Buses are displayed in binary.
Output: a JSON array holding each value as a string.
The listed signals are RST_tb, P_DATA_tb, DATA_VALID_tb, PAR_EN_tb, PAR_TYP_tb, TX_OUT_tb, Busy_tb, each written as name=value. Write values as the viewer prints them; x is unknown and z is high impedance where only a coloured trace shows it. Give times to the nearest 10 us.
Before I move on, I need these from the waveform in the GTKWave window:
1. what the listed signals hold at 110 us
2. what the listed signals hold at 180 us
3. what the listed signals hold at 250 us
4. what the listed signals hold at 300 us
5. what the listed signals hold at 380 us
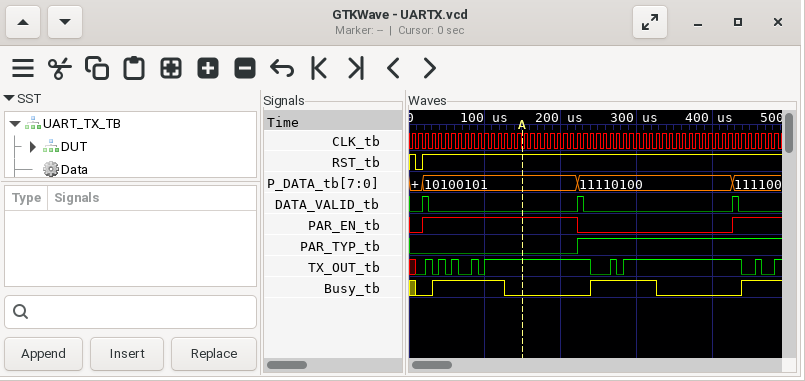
["RST_tb=1, P_DATA_tb=10100101, DATA_VALID_tb=0, PAR_EN_tb=1, PAR_TYP_tb=0, TX_OUT_tb=1, Busy_tb=1", "RST_tb=1, P_DATA_tb=10100101, DATA_VALID_tb=0, PAR_EN_tb=1, PAR_TYP_tb=0, TX_OUT_tb=1, Busy_tb=0", "RST_tb=1, P_DATA_tb=11110100, DATA_VALID_tb=0, PAR_EN_tb=0, PAR_TYP_tb=1, TX_OUT_tb=0, Busy_tb=1", "RST_tb=1, P_DATA_tb=11110100, DATA_VALID_tb=0, PAR_EN_tb=0, PAR_TYP_tb=1, TX_OUT_tb=1, Busy_tb=1", "RST_tb=1, P_DATA_tb=11110100, DATA_VALID_tb=0, PAR_EN_tb=0, PAR_TYP_tb=1, TX_OUT_tb=1, Busy_tb=0"]
